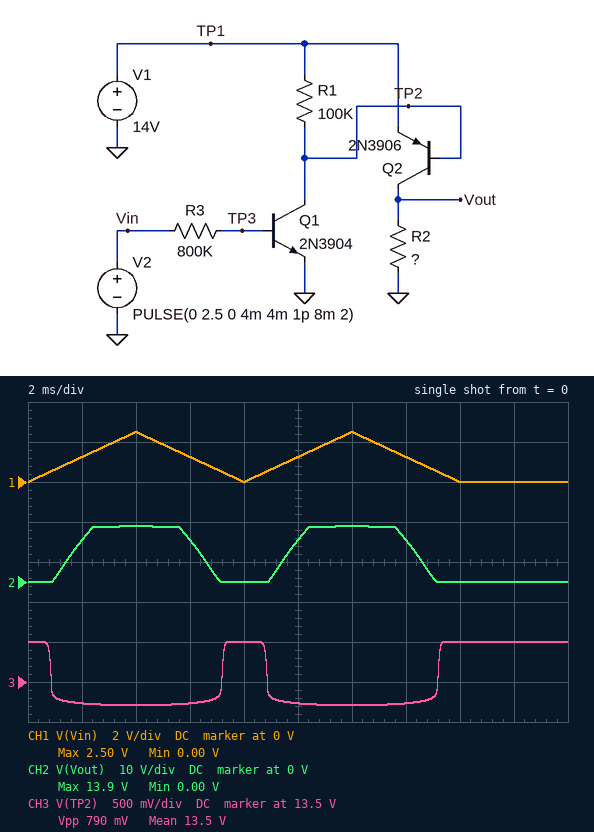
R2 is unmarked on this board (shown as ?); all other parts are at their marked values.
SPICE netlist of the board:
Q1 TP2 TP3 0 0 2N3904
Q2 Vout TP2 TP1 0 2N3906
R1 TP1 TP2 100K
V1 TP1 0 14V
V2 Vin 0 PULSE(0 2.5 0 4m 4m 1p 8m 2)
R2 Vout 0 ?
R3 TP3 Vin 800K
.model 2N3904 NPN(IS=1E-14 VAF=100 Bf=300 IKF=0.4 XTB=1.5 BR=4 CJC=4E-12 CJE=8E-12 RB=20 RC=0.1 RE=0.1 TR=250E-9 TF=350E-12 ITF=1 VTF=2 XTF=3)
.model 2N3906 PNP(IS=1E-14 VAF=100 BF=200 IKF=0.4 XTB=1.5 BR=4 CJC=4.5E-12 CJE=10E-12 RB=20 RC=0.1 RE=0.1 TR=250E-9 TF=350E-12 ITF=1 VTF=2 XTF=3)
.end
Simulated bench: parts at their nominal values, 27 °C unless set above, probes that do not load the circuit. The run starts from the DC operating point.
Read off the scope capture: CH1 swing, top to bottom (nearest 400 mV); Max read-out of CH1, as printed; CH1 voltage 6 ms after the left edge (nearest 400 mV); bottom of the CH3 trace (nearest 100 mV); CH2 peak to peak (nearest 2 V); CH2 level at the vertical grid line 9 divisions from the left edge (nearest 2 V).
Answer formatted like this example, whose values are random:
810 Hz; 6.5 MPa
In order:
2.4 V; 2.50 V; 1.2 V; 13.2 V; 14 V; 0 V
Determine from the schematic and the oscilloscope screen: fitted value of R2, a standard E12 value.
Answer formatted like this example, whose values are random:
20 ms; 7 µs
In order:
220 Ω
